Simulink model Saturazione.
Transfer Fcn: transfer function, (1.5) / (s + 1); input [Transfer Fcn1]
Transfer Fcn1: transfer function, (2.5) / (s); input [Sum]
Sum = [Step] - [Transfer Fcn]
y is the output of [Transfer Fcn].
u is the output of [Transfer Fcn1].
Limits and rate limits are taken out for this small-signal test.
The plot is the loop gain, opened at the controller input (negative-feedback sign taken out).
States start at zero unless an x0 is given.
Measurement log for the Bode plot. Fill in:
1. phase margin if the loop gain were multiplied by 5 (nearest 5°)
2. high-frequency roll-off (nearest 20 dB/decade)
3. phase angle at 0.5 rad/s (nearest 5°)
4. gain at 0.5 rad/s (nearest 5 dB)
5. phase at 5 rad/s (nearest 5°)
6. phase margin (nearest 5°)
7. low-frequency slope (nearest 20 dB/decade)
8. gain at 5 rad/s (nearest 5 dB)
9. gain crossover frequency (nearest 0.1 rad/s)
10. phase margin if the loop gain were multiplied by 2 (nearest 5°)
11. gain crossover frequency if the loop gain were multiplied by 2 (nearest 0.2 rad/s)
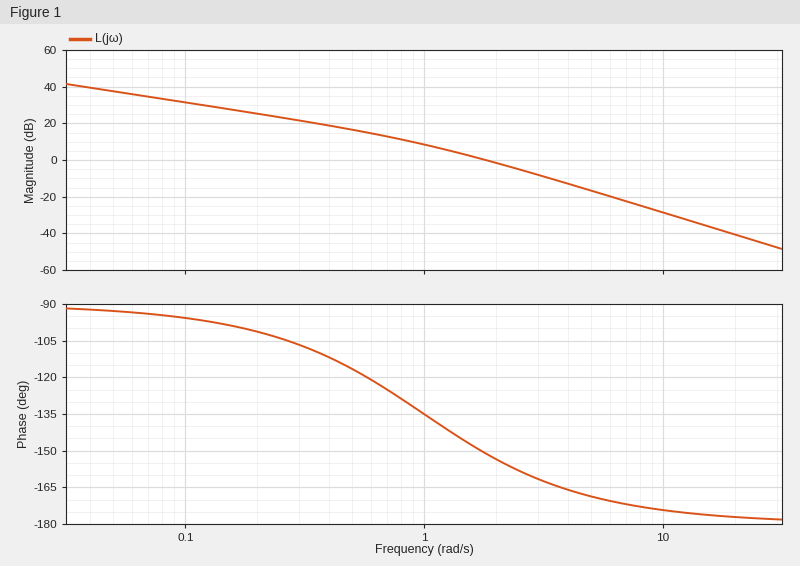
15°
-40 dB/decade
-115°
15 dB
-170°
30°
-20 dB/decade
-15 dB
1.8 rad/s
20°
2.6 rad/s
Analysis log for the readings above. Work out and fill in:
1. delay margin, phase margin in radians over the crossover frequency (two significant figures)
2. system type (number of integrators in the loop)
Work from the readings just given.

0.29 s
1
